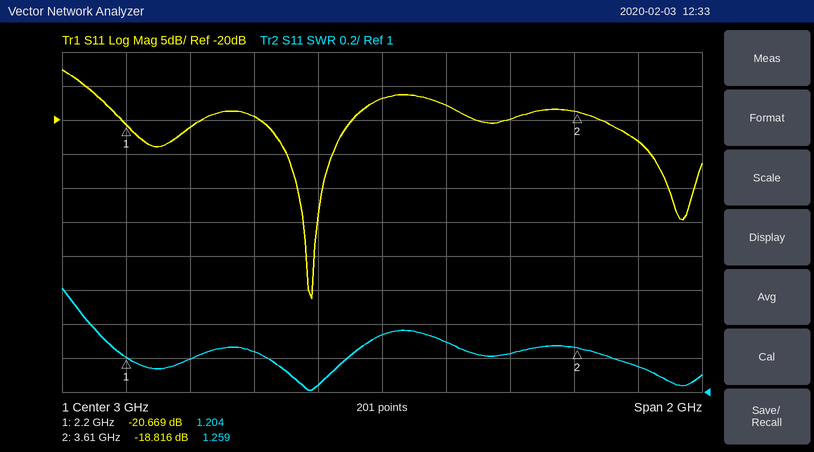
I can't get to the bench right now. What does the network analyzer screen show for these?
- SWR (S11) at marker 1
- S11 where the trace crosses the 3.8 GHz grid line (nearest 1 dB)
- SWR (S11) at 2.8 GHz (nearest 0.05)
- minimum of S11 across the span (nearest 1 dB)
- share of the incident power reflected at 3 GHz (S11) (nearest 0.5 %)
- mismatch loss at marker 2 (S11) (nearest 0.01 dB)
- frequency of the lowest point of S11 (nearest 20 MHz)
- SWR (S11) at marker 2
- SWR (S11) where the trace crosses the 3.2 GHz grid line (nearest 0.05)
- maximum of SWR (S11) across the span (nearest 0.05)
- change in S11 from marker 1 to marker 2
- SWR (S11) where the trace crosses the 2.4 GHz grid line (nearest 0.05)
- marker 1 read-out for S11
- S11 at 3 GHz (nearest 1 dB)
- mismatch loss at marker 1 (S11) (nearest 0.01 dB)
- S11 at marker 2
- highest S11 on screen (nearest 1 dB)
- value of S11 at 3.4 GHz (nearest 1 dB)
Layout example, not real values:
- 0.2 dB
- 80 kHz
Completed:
- 1.204
- -23 dB
- 1.05
- -46 dB
- 2.0 %
- 0.06 dB
- 2.78 GHz
- 1.259
- 1.30
- 1.60
- 1.853 dB
- 1.20
- -20.669 dB
- -17 dB
- 0.04 dB
- -18.816 dB
- -13 dB
- -20 dB
